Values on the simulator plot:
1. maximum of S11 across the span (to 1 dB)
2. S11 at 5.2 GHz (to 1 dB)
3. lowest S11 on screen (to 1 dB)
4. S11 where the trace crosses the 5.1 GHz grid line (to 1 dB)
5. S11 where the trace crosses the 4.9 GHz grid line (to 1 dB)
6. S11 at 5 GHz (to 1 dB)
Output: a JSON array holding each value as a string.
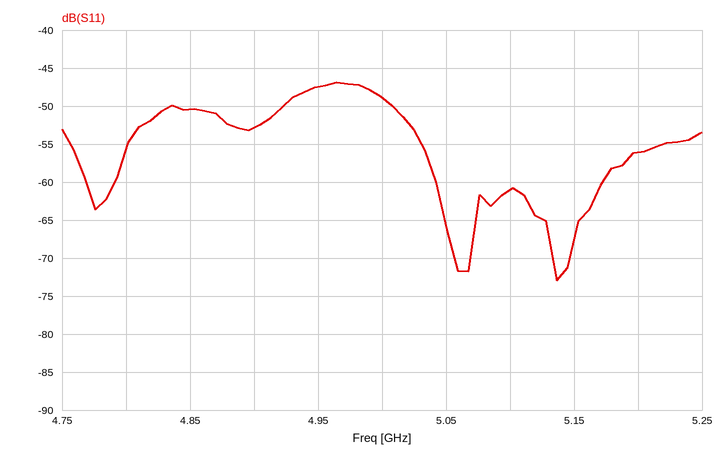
["-47 dB", "-56 dB", "-73 dB", "-61 dB", "-53 dB", "-49 dB"]
